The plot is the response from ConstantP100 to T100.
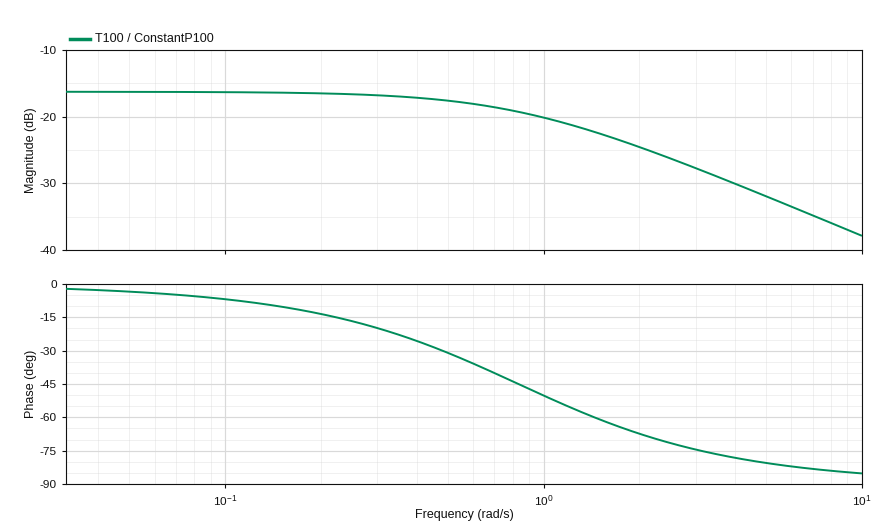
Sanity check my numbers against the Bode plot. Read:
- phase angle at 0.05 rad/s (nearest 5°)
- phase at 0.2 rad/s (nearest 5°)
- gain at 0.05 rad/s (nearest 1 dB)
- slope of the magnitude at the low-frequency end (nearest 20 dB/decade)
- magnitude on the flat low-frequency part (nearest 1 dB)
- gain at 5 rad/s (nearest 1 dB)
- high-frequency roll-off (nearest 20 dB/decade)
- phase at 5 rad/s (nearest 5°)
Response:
-5°
-15°
-16 dB
0 dB/decade
-16 dB
-32 dB
-20 dB/decade
-80°
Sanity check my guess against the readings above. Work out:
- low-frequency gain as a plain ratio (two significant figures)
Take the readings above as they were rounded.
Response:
0.16
